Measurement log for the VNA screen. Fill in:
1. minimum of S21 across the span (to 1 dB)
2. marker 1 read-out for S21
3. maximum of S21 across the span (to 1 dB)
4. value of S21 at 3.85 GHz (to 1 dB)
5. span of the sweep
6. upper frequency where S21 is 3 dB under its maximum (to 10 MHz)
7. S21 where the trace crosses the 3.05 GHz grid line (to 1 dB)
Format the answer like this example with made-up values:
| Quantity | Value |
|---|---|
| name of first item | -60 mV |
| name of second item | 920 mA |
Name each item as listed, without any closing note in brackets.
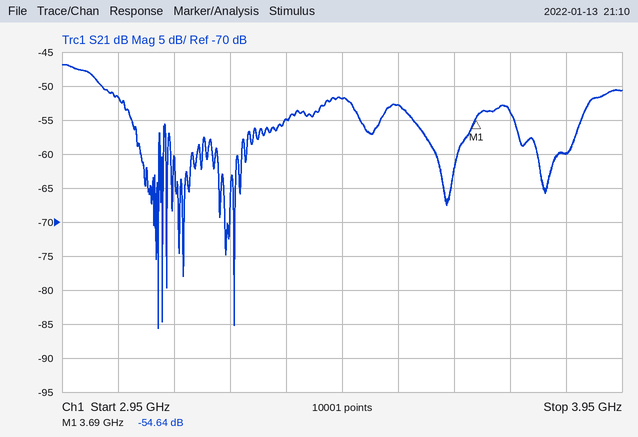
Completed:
| Quantity | Value |
|---|---|
| minimum of S21 across the span | -86 dB |
| marker 1 read-out for S21 | -54.64 dB |
| maximum of S21 across the span | -47 dB |
| value of S21 at 3.85 GHz | -60 dB |
| span of the sweep | 1 GHz |
| upper frequency where S21 is 3 dB under its maximum | 3.02 GHz |
| S21 where the trace crosses the 3.05 GHz grid line | -52 dB |
